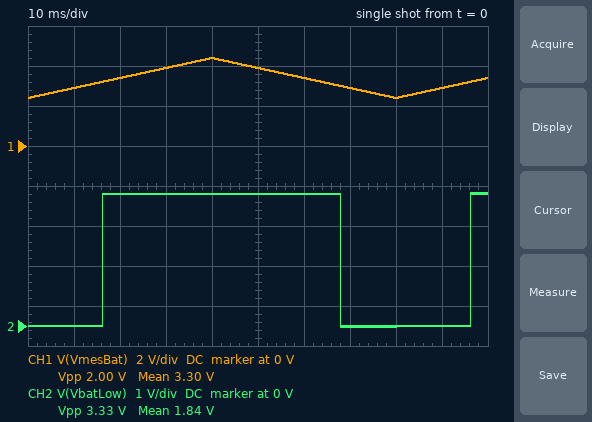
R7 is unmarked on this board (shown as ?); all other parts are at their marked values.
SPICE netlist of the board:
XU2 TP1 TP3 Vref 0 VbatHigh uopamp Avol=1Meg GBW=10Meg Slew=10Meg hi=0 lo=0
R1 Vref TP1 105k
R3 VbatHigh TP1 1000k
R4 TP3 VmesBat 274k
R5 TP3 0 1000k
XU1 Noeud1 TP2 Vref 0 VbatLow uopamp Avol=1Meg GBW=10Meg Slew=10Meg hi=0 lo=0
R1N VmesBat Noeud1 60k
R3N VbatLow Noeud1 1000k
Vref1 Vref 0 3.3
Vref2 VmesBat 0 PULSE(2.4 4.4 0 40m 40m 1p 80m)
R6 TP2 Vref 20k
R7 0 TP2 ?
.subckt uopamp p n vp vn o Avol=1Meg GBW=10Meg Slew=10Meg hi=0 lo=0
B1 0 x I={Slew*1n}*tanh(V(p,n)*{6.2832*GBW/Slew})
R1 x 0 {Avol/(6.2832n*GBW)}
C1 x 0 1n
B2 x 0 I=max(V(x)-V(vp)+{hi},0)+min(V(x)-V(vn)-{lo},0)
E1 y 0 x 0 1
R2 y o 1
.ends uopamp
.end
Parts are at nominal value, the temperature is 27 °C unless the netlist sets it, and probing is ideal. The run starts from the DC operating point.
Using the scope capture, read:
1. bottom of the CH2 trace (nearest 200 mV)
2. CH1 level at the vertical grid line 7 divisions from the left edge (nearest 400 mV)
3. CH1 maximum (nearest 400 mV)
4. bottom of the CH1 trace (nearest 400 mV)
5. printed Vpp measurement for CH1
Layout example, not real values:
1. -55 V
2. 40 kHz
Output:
1. 0 V
2. 2.8 V
3. 4.4 V
4. 2.4 V
5. 2.00 V
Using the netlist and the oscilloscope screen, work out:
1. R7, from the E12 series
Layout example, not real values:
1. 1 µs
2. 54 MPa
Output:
1. 220 kΩ
